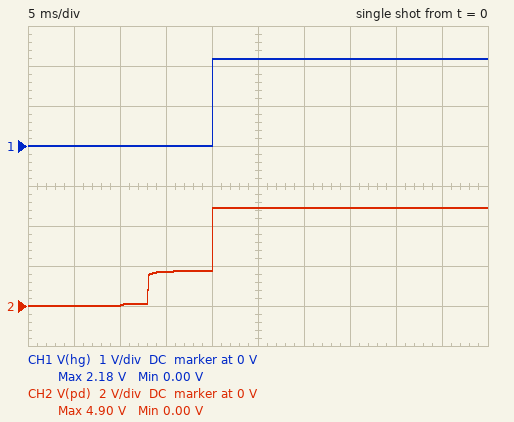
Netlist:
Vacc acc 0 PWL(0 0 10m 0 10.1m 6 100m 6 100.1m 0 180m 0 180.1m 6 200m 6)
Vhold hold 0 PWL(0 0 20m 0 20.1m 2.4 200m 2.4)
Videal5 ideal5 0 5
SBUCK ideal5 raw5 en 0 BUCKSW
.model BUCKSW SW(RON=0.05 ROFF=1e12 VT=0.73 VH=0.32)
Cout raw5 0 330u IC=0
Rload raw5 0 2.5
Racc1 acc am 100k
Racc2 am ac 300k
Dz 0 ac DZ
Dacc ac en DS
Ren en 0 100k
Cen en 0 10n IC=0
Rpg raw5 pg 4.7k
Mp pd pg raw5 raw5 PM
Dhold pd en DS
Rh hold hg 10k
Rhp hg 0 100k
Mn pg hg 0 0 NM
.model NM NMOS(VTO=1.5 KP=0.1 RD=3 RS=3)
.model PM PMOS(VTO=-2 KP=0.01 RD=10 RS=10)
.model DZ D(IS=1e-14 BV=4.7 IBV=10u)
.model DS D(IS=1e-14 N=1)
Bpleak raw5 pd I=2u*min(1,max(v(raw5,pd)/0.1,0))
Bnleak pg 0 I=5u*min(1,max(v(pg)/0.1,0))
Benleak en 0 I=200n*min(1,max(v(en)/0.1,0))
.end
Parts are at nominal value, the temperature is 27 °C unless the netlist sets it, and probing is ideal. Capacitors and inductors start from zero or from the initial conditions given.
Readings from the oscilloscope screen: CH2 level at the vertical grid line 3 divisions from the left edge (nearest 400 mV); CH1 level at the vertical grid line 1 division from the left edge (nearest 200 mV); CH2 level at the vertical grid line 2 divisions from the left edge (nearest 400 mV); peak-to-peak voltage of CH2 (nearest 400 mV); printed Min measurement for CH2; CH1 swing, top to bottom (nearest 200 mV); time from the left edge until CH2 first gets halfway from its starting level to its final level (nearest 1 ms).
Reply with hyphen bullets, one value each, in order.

- 1.6 V
- 0 V
- 0 V
- 4.8 V
- 0.00 V
- 2.2 V
- 20 ms
